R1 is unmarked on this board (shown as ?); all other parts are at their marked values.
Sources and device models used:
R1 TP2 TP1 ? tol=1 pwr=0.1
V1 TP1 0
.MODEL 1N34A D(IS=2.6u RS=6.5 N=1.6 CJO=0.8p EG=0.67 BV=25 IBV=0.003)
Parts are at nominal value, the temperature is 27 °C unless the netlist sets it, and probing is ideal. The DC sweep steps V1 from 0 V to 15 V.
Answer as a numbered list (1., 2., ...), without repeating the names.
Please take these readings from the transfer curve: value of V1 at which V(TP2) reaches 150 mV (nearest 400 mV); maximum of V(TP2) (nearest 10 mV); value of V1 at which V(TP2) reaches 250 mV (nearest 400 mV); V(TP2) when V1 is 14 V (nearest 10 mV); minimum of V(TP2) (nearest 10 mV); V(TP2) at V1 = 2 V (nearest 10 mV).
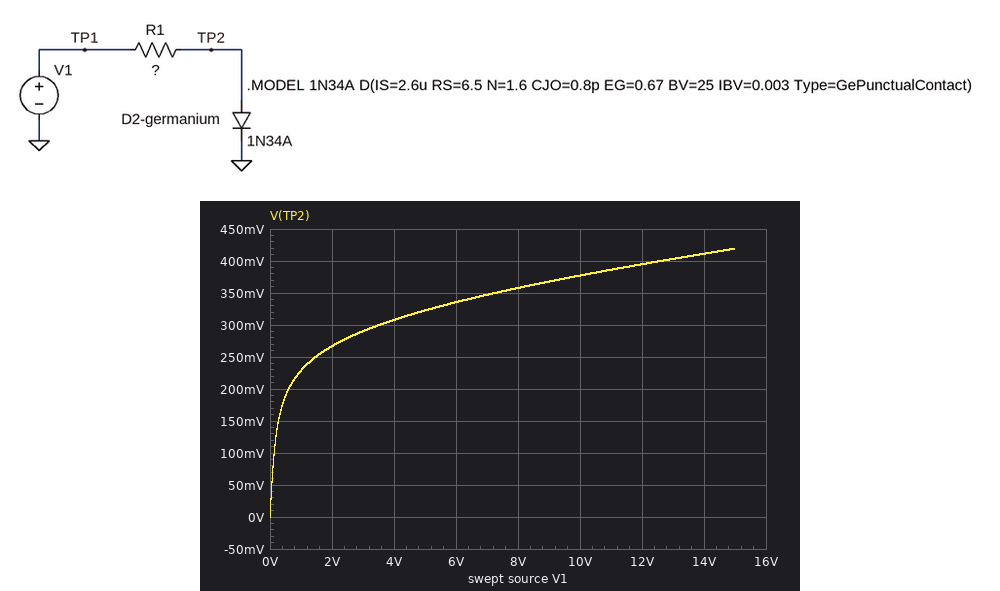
1. 400 mV
2. 420 mV
3. 1.6 V
4. 410 mV
5. 0 V
6. 270 mV
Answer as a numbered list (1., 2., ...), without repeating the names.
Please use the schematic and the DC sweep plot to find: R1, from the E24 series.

1. 1.3 kΩ
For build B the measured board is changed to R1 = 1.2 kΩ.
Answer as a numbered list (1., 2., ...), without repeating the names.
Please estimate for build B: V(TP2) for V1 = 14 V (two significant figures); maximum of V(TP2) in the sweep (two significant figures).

1. 420 mV
2. 430 mV
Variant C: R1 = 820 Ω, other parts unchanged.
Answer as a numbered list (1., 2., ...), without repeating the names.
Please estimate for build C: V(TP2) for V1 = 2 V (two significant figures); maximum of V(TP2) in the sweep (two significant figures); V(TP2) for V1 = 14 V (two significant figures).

1. 290 mV
2. 480 mV
3. 470 mV
